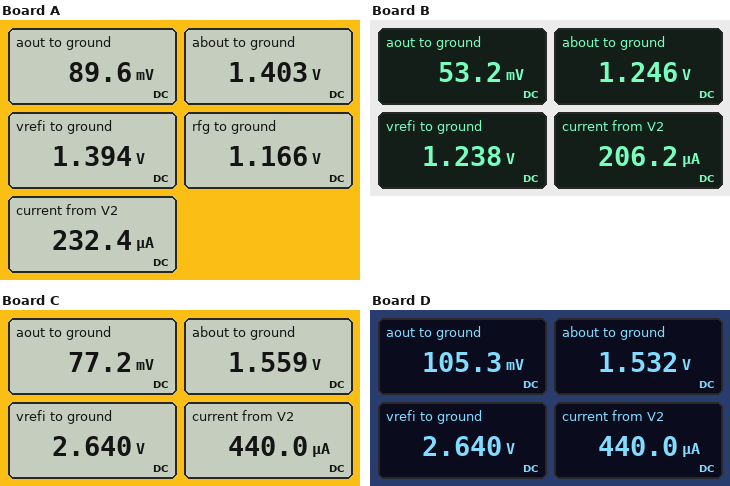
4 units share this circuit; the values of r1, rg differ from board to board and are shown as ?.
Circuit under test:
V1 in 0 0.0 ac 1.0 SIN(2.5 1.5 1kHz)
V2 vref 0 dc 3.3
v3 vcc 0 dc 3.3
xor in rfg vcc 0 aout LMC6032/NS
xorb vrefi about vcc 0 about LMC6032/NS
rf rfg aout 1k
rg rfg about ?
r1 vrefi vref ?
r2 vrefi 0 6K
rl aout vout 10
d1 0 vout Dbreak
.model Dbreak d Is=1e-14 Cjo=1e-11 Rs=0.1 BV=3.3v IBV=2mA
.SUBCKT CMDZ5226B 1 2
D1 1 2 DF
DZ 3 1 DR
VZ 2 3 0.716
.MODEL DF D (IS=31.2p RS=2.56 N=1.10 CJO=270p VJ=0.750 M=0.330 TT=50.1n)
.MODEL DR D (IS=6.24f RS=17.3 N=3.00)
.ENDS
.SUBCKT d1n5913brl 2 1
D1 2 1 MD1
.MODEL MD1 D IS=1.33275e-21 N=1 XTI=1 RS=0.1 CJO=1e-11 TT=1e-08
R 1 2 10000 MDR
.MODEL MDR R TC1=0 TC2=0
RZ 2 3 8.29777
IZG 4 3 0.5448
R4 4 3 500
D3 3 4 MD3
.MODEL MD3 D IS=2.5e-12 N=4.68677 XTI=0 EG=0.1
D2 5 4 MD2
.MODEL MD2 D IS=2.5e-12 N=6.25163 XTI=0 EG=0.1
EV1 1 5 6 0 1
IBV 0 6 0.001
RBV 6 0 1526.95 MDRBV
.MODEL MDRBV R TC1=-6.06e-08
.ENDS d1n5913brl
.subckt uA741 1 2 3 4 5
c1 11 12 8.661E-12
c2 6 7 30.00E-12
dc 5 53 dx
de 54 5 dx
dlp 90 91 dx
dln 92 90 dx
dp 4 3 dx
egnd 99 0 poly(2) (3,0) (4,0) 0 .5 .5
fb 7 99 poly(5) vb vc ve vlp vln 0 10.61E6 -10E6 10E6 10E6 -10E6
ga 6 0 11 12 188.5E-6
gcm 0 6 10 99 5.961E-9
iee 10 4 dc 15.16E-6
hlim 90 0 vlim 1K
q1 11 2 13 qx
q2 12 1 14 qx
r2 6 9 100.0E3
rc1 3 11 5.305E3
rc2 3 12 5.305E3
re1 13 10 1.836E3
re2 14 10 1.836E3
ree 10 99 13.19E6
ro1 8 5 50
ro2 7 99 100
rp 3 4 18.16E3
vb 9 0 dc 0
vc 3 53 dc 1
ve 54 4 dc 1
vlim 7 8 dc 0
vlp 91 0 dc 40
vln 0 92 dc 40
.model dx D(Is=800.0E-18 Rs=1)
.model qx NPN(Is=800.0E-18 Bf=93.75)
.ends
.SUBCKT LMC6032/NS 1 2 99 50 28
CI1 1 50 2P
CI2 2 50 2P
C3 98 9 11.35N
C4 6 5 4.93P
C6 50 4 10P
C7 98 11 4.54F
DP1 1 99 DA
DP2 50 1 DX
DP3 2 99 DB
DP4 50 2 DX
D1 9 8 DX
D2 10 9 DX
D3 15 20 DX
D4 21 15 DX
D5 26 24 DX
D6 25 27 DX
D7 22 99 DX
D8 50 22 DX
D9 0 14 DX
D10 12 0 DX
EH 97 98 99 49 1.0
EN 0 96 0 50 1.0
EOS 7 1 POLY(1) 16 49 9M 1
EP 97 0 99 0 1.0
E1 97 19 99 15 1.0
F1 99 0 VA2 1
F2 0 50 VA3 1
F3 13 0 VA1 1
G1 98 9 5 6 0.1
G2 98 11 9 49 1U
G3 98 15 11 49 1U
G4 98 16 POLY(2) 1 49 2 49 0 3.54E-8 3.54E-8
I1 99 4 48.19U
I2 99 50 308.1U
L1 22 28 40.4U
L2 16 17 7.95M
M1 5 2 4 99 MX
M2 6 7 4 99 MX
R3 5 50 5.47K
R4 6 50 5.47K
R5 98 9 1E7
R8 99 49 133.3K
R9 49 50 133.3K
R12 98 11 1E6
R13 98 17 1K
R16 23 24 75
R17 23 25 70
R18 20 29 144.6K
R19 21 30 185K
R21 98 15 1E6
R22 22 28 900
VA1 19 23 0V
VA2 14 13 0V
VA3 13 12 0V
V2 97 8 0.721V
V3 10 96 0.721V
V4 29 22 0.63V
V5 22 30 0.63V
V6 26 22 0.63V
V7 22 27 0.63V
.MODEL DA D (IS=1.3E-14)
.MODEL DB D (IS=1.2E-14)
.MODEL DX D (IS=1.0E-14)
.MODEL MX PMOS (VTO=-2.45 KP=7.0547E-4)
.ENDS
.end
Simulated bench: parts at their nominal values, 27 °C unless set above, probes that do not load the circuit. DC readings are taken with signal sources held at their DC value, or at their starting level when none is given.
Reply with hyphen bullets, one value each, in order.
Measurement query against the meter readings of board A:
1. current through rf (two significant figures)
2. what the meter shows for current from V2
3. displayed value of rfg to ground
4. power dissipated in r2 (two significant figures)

- 1.1 mA
- 232.4 µA
- 1.166 V
- 320 µW
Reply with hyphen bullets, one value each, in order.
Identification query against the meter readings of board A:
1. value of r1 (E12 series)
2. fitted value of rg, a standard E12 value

- 8.2 kΩ
- 220 Ω
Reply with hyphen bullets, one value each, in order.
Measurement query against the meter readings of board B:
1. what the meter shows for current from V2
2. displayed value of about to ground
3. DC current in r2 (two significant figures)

- 206.2 µA
- 1.246 V
- 210 µA
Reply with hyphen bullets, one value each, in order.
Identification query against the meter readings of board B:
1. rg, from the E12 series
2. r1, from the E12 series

- 680 Ω
- 10 kΩ
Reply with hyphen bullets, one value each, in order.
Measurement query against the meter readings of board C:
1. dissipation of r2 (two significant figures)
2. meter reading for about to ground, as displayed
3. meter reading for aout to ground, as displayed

- 1.2 mW
- 1.559 V
- 77.2 mV
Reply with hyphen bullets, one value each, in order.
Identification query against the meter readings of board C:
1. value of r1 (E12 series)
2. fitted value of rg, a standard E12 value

- 1.5 kΩ
- 560 Ω
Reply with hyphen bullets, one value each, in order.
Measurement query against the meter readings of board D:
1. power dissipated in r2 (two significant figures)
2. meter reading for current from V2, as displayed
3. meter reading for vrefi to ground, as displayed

- 1.2 mW
- 440.0 µA
- 2.640 V
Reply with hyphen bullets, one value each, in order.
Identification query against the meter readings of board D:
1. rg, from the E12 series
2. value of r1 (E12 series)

- 150 Ω
- 1.5 kΩ
